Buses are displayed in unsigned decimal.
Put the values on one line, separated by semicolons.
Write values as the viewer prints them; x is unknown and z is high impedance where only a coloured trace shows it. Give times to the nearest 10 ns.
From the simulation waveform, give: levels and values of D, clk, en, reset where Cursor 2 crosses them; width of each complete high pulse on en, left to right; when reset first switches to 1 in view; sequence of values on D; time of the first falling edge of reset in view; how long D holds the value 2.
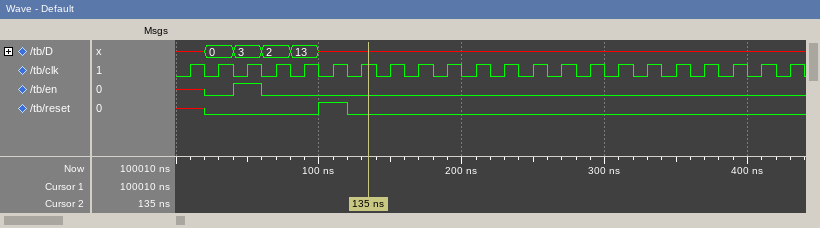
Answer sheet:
D=x, clk=1, en=0, reset=0; 20 ns; 100 ns; x, 0, 3, 2, 13, x; 120 ns; 20 ns
